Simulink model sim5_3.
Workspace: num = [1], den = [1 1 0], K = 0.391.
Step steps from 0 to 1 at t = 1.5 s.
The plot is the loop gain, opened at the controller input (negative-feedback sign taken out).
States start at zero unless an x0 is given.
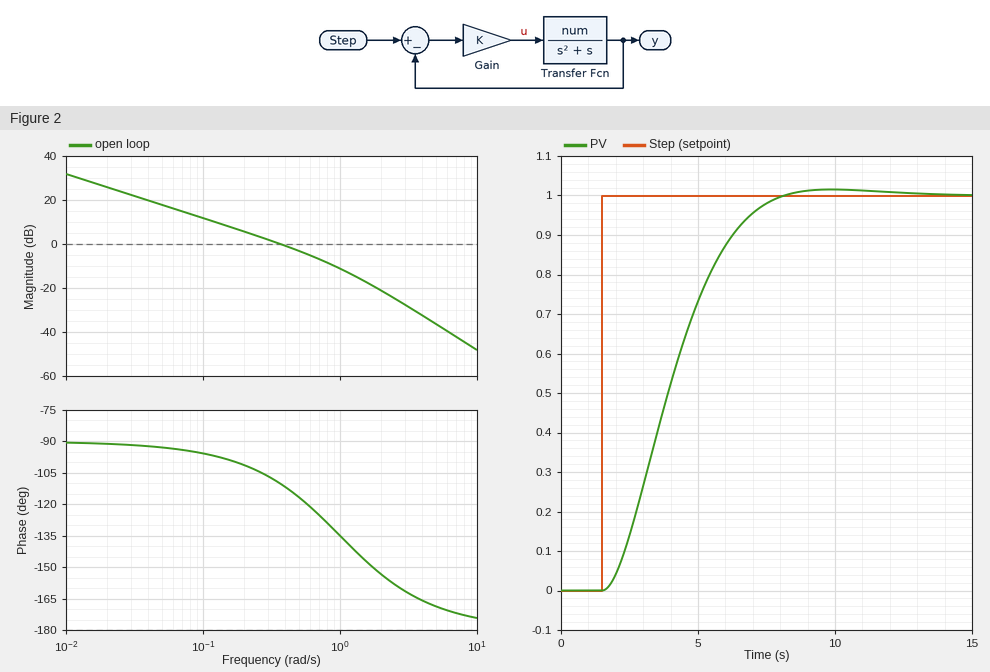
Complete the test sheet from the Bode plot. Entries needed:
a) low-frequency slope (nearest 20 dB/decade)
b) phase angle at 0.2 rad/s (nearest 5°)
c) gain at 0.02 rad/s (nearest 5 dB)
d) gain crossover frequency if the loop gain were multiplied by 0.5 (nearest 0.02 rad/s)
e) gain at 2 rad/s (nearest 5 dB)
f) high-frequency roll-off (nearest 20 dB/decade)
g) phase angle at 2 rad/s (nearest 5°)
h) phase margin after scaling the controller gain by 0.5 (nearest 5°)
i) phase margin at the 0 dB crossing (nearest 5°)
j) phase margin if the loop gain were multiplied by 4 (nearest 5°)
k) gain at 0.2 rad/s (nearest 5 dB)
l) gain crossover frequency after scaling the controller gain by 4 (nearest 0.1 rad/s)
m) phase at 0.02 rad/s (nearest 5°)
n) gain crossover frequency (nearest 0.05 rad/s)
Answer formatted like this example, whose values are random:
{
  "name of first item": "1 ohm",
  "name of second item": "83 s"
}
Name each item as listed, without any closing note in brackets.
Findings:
{
  "low-frequency slope": "-20 dB/decade",
  "phase angle at 0.2 rad/s": "-100°",
  "gain at 0.02 rad/s": "25 dB",
  "gain crossover frequency if the loop gain were multiplied by 0.5": "0.20 rad/s",
  "gain at 2 rad/s": "-20 dB",
  "high-frequency roll-off": "-40 dB/decade",
  "phase angle at 2 rad/s": "-155°",
  "phase margin after scaling the controller gain by 0.5": "80°",
  "phase margin at the 0 dB crossing": "70°",
  "phase margin if the loop gain were multiplied by 4": "45°",
  "gain at 0.2 rad/s": "5 dB",
  "gain crossover frequency after scaling the controller gain by 4": "1.1 rad/s",
  "phase at 0.02 rad/s": "-90°",
  "gain crossover frequency": "0.35 rad/s"
}
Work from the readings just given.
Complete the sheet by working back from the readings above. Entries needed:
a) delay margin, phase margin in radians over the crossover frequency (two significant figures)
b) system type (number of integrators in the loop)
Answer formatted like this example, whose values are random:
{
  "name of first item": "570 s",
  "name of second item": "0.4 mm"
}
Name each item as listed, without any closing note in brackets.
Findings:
{
  "delay margin, phase margin in radians over the crossover frequency": "3.5 s",
  "system type": "1"
}
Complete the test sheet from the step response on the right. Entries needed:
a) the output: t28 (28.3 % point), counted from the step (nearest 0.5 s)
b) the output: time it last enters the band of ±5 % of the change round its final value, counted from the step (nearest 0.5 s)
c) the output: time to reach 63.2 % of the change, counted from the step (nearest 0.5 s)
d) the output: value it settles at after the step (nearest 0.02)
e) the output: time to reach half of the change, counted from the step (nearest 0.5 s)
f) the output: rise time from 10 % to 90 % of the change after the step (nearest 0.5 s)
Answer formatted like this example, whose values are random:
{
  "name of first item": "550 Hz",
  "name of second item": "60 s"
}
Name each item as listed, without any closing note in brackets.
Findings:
{
  "the output: t28 (28.3 % point), counted from the step": "1.5 s",
  "the output: time it last enters the band of ±5 % of the change round its final value, counted from the step": "5.5 s",
  "the output: time to reach 63.2 % of the change, counted from the step": "3.0 s",
  "the output: value it settles at after the step": "1.00",
  "the output: time to reach half of the change, counted from the step": "2.5 s",
  "the output: rise time from 10 % to 90 % of the change after the step": "4.0 s"
}
